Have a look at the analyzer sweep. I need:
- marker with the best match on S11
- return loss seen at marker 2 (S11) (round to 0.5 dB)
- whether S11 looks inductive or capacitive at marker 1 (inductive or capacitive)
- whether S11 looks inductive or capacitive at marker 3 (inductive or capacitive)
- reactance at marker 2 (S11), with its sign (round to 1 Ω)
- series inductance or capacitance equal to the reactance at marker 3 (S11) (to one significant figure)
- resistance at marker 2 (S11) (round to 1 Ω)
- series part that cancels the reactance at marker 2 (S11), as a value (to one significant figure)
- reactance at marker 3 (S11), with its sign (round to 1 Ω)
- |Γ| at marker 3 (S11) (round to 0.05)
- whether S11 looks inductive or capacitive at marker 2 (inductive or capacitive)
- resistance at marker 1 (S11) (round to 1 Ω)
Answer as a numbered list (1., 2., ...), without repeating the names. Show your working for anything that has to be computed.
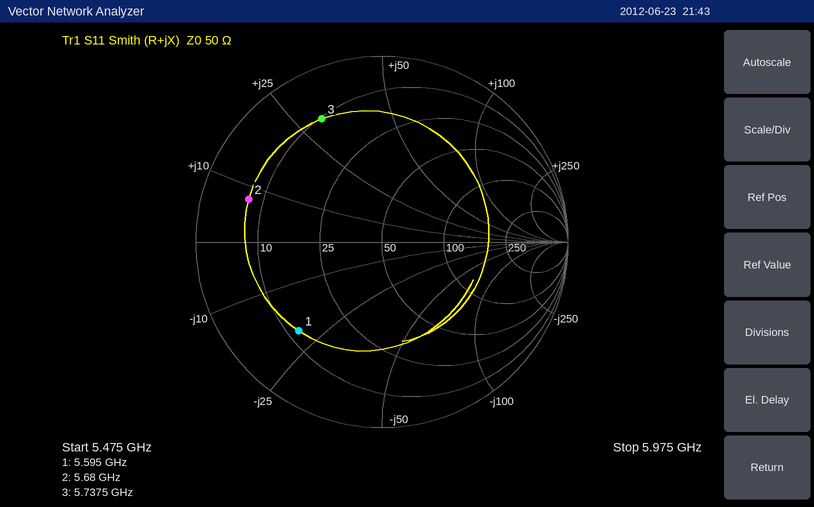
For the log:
1. marker 1
2. 2.5 dB
3. capacitive
4. inductive
5. +8 Ω
6. L = 30 Ω/(2π × 5.7375 GHz) ≈ 832 pH, so 800 pH to one significant figure
7. 7 Ω
8. C = 1/(2π × 5.68 GHz × 8 Ω) ≈ 4 pF
9. +30 Ω
10. 0.75
11. inductive
12. 12 Ω
